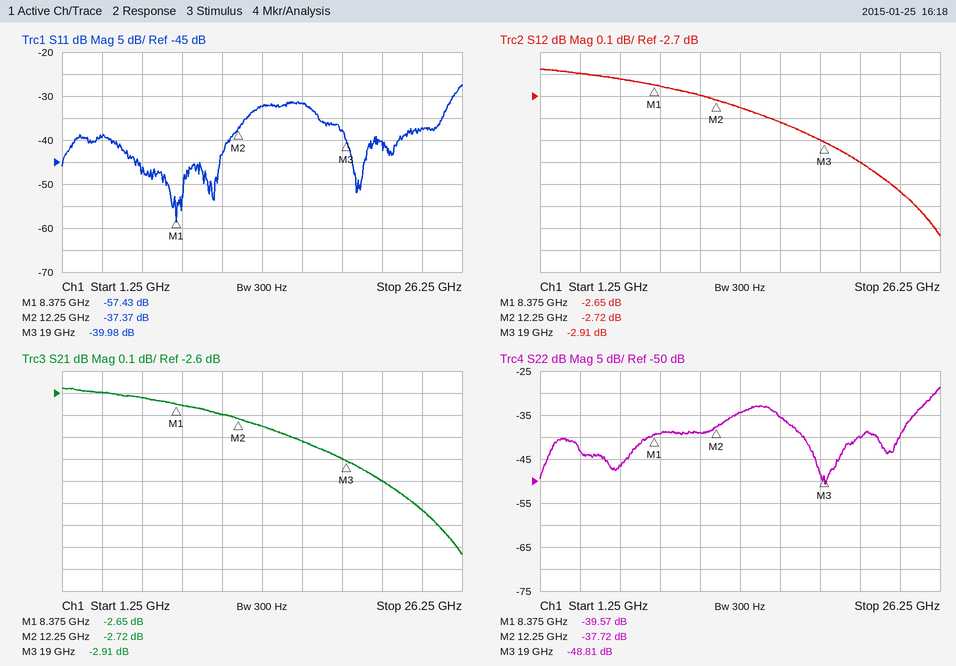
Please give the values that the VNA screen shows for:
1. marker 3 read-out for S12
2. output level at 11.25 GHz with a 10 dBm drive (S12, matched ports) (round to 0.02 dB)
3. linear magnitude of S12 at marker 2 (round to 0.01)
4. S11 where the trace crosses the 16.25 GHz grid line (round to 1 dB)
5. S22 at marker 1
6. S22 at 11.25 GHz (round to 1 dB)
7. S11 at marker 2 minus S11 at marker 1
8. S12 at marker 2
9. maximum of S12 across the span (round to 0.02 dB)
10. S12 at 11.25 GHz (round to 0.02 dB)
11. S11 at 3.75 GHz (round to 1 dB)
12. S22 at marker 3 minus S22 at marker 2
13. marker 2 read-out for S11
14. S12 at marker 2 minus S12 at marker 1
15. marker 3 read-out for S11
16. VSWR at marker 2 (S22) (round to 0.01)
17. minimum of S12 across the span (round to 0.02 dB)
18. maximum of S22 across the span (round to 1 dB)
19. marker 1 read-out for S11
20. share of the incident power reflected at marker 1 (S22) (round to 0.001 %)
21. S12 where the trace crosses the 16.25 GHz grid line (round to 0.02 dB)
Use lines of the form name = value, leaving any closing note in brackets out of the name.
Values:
marker 3 read-out for S12 = -2.91 dB
output level at 11.25 GHz with a 10 dBm drive (S12, matched ports) = 7.30 dBm
linear magnitude of S12 at marker 2 = 0.73
S11 where the trace crosses the 16.25 GHz grid line = -32 dB
S22 at marker 1 = -39.57 dB
S22 at 11.25 GHz = -39 dB
S11 at marker 2 minus S11 at marker 1 = 20.06 dB
S12 at marker 2 = -2.72 dB
maximum of S12 across the span = -2.58 dB
S12 at 11.25 GHz = -2.70 dB
S11 at 3.75 GHz = -39 dB
S22 at marker 3 minus S22 at marker 2 = -11.09 dB
marker 2 read-out for S11 = -37.37 dB
S12 at marker 2 minus S12 at marker 1 = -0.07 dB
marker 3 read-out for S11 = -39.98 dB
VSWR at marker 2 (S22) = 1.03
minimum of S12 across the span = -3.34 dB
maximum of S22 across the span = -29 dB
marker 1 read-out for S11 = -57.43 dB
share of the incident power reflected at marker 1 (S22) = 0.011 %
S12 where the trace crosses the 16.25 GHz grid line = -2.82 dB
